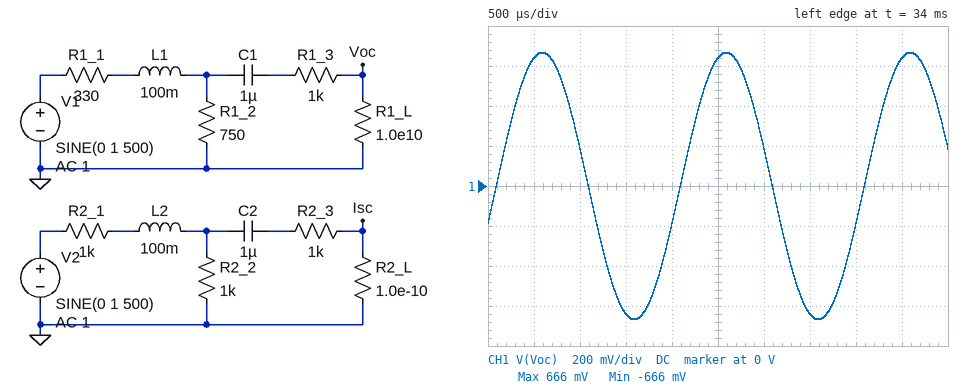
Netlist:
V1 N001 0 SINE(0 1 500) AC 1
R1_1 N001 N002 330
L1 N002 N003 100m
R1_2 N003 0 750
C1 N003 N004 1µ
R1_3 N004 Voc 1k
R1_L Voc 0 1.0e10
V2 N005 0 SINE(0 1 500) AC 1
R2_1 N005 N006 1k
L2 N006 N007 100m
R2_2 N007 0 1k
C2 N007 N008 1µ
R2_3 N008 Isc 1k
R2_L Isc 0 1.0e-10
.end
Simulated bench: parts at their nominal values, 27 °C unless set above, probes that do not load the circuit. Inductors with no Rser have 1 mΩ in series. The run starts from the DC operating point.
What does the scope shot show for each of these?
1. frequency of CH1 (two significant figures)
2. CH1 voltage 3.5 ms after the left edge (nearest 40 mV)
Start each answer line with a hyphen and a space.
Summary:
- 500 Hz
- -640 mV
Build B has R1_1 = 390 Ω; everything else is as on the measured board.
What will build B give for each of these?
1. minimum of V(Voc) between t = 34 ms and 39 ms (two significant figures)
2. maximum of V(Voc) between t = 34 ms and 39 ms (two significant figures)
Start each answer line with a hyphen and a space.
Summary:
- -630 mV
- 630 mV
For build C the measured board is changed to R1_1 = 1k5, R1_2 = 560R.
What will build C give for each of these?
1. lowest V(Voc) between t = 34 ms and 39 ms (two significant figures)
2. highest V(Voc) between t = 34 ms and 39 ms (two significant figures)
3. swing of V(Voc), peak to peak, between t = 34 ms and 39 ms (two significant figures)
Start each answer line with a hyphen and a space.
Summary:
- -270 mV
- 270 mV
- 540 mV
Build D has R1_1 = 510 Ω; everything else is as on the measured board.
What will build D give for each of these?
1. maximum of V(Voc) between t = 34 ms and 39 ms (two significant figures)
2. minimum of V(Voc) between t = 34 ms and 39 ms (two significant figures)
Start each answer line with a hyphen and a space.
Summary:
- 580 mV
- -580 mV
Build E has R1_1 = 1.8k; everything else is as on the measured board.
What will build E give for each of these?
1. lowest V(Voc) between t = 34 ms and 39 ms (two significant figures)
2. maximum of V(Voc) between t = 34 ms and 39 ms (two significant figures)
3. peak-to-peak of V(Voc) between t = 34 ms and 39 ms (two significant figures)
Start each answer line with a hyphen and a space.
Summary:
- -290 mV
- 290 mV
- 580 mV
